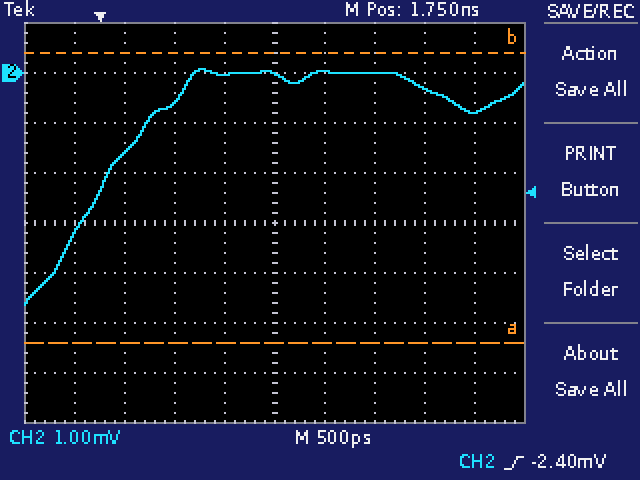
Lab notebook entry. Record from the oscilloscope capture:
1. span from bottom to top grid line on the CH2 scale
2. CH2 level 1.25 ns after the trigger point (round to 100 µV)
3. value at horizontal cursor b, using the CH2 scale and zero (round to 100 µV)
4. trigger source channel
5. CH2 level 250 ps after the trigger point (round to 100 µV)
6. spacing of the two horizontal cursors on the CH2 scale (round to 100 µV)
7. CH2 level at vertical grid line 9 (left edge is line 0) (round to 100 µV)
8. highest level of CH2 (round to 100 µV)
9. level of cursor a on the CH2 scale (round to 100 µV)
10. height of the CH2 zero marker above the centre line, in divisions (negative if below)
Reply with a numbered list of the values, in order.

1. 8 mV
2. 0.0 mV
3. 400 µV
4. CH2
5. -1.6 mV
6. 5.8 mV
7. -800 µV
8. 100 µV
9. -5.4 mV
10. +3.0 div
